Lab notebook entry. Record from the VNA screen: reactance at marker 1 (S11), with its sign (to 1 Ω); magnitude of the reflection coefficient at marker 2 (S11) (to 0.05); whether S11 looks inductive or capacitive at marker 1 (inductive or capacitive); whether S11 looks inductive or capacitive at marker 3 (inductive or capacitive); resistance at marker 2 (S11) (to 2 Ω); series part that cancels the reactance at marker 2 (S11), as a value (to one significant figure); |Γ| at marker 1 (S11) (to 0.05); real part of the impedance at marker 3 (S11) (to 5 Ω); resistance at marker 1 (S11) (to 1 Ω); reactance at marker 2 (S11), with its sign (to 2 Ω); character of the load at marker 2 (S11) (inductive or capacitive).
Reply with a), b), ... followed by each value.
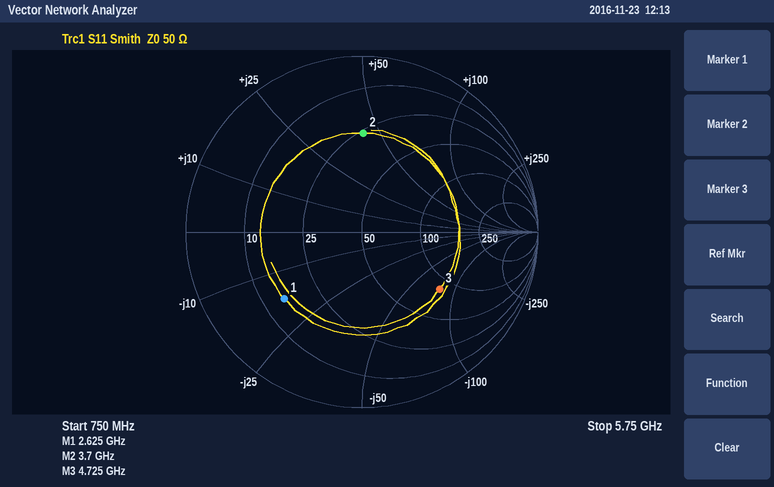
a) -17 Ω
b) 0.55
c) capacitive
d) capacitive
e) 26 Ω
f) 1.0 pF
g) 0.60
h) 85 Ω
i) 15 Ω
j) +44 Ω
k) inductive
